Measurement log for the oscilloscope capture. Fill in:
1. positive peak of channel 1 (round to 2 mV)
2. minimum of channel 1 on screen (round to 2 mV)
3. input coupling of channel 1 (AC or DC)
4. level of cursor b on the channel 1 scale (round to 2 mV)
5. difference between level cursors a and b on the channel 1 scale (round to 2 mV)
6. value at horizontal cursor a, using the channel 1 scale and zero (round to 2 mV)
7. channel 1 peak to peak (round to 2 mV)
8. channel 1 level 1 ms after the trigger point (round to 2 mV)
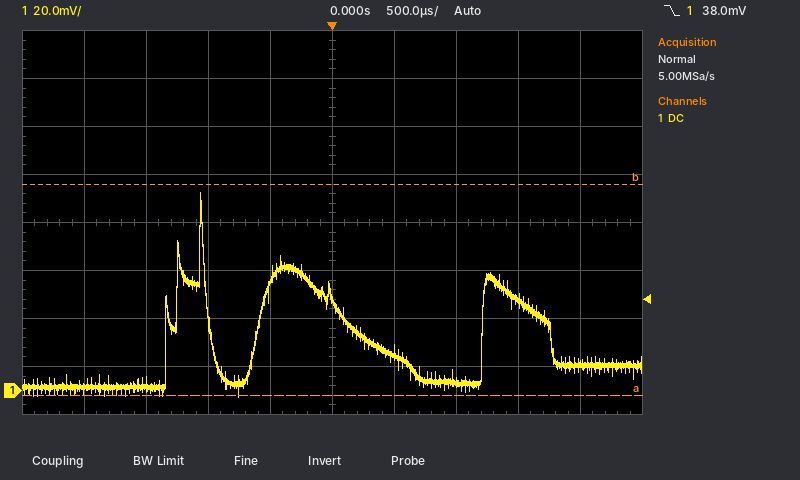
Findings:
82 mV
-2 mV
DC
86 mV
88 mV
-2 mV
84 mV
4 mV
